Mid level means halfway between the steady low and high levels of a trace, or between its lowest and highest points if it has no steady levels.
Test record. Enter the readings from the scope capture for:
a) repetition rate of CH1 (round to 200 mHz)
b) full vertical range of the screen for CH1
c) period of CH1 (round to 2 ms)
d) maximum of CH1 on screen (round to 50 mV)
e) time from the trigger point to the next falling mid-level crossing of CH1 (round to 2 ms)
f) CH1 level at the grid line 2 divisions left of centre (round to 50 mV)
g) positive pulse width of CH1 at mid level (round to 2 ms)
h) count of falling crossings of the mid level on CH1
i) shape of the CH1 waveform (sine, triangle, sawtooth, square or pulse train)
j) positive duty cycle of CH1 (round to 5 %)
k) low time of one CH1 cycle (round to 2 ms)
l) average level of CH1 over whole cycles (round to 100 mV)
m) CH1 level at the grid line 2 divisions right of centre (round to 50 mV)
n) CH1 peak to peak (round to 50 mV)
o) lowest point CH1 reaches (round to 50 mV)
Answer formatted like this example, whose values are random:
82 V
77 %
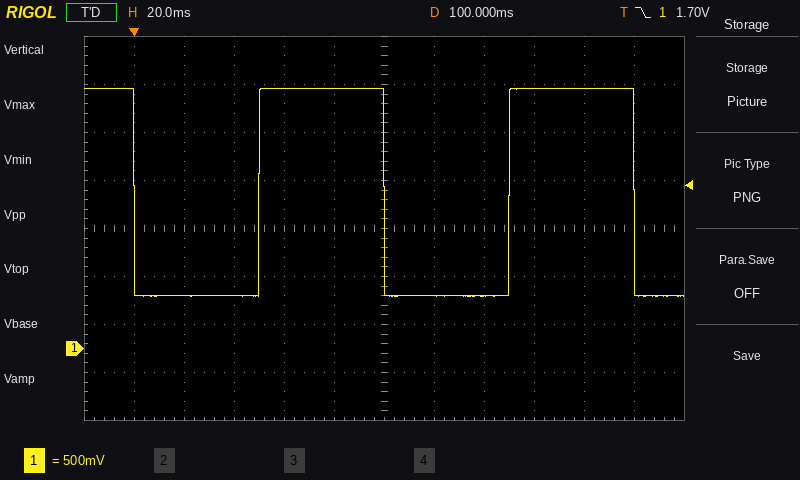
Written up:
10.0 Hz
4 V
100 ms
2.70 V
100 ms
2.70 V
50 ms
3
square
50 %
50 ms
1.6 V
550 mV
2.15 V
550 mV
